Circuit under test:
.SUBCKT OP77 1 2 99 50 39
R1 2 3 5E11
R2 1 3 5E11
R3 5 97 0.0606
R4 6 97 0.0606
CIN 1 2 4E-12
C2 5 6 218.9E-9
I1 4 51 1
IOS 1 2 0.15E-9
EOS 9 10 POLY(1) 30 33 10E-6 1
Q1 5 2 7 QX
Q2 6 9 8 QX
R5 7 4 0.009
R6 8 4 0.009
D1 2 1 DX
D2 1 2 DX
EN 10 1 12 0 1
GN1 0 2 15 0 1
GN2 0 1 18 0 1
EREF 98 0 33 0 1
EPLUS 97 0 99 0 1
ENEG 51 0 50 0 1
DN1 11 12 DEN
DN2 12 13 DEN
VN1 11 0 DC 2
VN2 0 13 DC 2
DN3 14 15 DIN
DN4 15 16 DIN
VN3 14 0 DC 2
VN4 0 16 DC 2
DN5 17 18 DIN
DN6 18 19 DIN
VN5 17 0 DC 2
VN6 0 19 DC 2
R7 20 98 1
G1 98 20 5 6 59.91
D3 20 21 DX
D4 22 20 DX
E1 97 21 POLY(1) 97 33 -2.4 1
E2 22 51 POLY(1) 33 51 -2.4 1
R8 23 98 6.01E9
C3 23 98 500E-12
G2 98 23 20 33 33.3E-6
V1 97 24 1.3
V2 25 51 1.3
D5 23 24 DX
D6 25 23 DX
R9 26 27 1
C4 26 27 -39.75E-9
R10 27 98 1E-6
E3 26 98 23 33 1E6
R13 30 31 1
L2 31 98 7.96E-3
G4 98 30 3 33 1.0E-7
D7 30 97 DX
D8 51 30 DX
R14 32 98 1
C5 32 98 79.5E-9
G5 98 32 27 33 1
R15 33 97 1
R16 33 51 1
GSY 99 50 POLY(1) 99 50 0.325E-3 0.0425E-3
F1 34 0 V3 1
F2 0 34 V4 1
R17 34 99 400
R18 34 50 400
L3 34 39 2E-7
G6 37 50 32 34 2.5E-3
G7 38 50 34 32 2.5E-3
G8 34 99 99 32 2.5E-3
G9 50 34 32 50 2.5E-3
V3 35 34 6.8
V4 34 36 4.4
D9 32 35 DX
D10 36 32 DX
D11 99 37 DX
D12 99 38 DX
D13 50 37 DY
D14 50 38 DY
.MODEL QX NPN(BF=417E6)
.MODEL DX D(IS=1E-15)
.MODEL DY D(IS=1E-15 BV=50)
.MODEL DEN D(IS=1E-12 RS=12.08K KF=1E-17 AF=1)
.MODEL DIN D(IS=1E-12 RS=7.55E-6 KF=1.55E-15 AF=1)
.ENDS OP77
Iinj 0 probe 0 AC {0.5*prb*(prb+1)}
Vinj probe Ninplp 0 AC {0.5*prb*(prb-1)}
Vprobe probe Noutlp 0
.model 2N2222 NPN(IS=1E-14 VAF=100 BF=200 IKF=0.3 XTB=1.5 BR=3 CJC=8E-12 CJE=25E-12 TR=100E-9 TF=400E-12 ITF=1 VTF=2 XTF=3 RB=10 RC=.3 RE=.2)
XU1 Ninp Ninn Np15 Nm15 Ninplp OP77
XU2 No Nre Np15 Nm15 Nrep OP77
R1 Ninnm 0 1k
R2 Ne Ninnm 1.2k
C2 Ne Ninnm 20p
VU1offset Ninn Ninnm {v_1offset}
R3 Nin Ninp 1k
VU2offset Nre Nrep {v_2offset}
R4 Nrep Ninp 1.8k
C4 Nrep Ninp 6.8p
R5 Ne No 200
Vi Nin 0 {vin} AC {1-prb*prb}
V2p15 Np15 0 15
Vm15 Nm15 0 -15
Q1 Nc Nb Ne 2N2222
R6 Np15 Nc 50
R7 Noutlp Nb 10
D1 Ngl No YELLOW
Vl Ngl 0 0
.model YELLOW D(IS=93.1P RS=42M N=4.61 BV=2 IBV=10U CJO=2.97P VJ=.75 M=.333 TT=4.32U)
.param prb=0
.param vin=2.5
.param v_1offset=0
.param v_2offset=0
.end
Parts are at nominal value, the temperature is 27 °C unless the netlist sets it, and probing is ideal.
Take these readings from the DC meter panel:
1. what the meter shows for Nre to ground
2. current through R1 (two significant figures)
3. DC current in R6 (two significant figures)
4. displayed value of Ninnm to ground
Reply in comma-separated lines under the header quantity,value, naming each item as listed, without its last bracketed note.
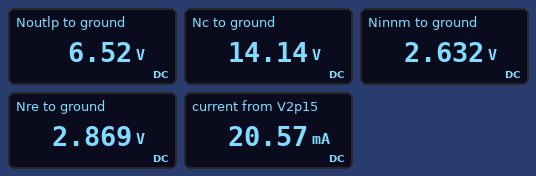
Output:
quantity,value
what the meter shows for Nre to ground,2.869 V
current through R1,2.6 mA
DC current in R6,17 mA
displayed value of Ninnm to ground,2.632 V
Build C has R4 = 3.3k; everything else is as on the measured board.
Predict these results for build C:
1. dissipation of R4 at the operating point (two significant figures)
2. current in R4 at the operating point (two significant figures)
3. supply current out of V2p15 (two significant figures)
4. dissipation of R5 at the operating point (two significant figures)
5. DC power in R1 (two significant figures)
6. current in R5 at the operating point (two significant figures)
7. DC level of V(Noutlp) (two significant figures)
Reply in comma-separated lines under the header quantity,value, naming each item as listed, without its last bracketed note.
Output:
quantity,value
dissipation of R4 at the operating point,24 µW
current in R4 at the operating point,85 µA
supply current out of V2p15,20 mA
dissipation of R5 at the operating point,40 mW
DC power in R1,6.7 mW
current in R5 at the operating point,14 mA
DC level of V(Noutlp),6.4 V
